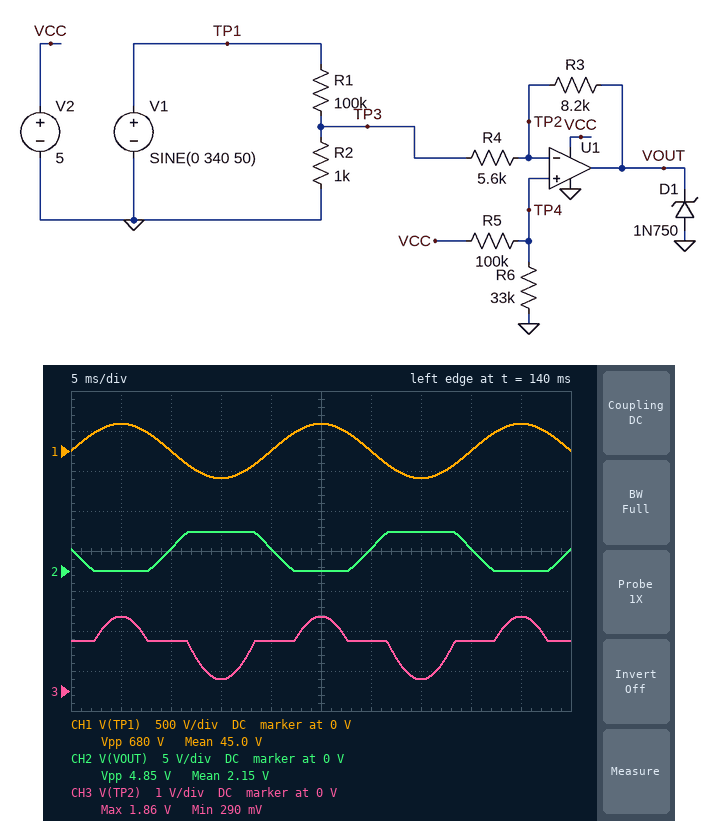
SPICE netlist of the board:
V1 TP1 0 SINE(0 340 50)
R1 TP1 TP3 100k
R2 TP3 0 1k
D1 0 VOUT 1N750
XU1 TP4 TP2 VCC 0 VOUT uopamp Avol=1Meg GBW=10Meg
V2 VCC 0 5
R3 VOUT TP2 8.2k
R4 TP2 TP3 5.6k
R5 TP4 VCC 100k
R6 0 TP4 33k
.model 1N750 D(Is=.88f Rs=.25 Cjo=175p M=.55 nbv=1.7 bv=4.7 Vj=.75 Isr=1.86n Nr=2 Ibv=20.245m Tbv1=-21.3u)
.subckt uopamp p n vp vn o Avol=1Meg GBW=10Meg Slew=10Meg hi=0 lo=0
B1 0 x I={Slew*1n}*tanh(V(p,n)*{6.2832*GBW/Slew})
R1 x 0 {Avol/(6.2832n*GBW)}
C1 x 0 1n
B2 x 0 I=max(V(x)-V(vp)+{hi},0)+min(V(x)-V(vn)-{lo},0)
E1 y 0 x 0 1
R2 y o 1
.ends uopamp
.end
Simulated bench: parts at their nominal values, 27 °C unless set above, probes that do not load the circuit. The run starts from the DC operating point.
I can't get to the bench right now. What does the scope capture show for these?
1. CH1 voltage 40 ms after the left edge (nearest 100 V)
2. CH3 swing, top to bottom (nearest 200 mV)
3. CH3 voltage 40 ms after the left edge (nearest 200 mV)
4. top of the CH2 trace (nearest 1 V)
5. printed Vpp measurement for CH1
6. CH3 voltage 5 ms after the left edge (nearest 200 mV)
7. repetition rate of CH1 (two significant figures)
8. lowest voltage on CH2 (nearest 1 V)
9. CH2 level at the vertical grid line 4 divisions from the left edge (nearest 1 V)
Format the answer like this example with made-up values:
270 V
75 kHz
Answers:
0 V
1.6 V
1.2 V
5 V
680 V
1.8 V
50 Hz
0 V
3 V
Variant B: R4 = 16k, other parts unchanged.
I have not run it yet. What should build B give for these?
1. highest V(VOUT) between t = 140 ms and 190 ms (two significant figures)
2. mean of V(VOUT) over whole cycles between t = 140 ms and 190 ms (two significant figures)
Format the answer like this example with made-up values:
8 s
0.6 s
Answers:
3.5 V
1.8 V
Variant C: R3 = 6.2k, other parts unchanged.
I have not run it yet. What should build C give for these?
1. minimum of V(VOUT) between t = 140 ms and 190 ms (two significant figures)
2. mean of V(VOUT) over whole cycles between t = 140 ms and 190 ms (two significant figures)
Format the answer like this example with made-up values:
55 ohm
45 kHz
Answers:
-9.6 mV
2.4 V
